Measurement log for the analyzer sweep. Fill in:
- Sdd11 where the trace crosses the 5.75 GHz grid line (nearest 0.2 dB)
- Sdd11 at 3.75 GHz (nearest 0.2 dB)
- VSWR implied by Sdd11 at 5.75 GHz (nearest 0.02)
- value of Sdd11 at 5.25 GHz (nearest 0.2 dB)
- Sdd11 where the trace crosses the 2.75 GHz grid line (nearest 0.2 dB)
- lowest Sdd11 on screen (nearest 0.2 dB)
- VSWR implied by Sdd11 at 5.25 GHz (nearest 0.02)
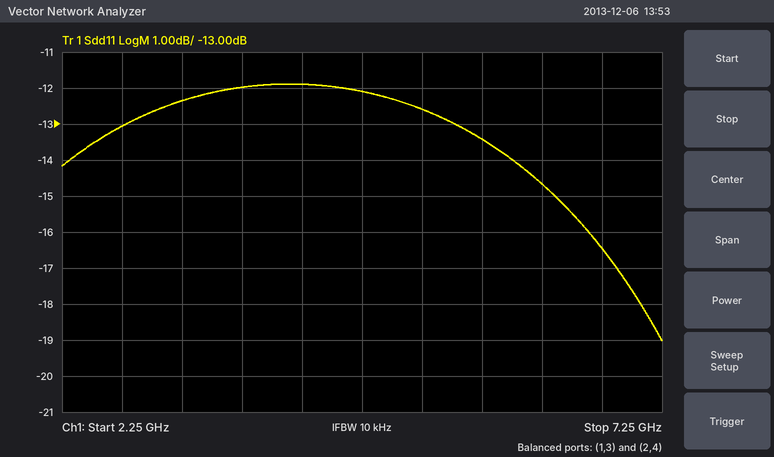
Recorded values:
-13.4 dB
-12.0 dB
1.54
-12.6 dB
-13.0 dB
-19.0 dB
1.62
